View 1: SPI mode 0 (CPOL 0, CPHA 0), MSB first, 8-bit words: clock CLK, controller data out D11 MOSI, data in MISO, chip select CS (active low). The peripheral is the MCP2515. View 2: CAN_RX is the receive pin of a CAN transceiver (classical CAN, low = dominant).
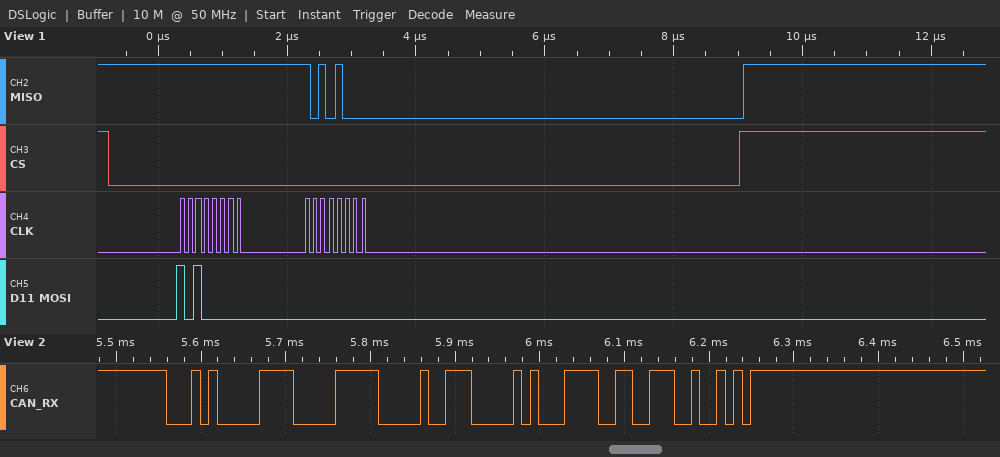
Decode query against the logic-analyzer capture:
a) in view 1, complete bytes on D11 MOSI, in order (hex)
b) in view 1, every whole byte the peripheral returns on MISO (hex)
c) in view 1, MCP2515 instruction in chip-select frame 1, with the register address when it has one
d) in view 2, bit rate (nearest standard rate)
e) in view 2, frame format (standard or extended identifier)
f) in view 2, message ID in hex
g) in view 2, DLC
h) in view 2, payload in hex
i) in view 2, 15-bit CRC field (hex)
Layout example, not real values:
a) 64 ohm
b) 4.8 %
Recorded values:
a) A0 00
b) FF A8
c) READ STATUS
d) 100 kbit/s
e) extended
f) 0x05041E07
g) 1
h) 1E
i) 0x3392
